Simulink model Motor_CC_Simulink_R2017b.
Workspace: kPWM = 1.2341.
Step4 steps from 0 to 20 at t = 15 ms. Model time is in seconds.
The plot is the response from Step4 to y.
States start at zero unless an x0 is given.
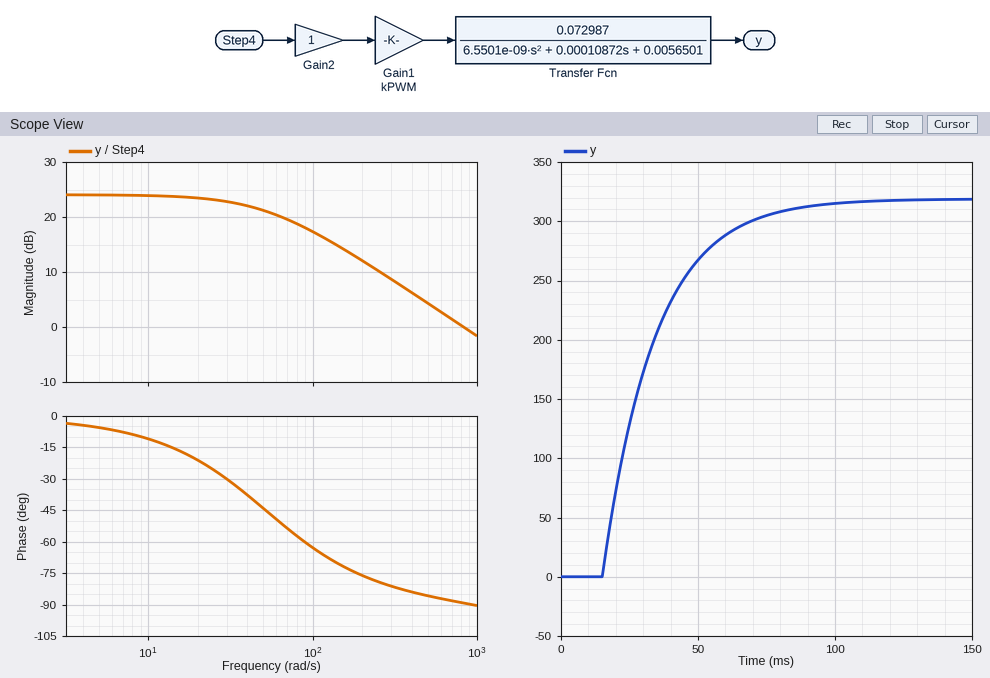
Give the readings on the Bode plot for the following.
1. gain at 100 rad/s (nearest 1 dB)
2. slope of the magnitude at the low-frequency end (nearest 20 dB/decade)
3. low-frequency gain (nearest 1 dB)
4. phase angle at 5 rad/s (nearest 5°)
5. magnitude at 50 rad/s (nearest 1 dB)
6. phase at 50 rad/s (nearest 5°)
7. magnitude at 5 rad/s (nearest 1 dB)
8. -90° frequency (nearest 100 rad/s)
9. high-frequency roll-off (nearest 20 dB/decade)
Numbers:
17 dB
0 dB/decade
24 dB
-5°
21 dB
-45°
24 dB
900 rad/s
-20 dB/decade
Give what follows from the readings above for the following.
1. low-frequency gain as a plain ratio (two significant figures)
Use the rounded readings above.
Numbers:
16
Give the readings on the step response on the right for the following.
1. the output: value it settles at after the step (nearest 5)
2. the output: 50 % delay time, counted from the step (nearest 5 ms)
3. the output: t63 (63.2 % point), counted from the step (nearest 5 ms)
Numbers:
320
15 ms
20 ms
